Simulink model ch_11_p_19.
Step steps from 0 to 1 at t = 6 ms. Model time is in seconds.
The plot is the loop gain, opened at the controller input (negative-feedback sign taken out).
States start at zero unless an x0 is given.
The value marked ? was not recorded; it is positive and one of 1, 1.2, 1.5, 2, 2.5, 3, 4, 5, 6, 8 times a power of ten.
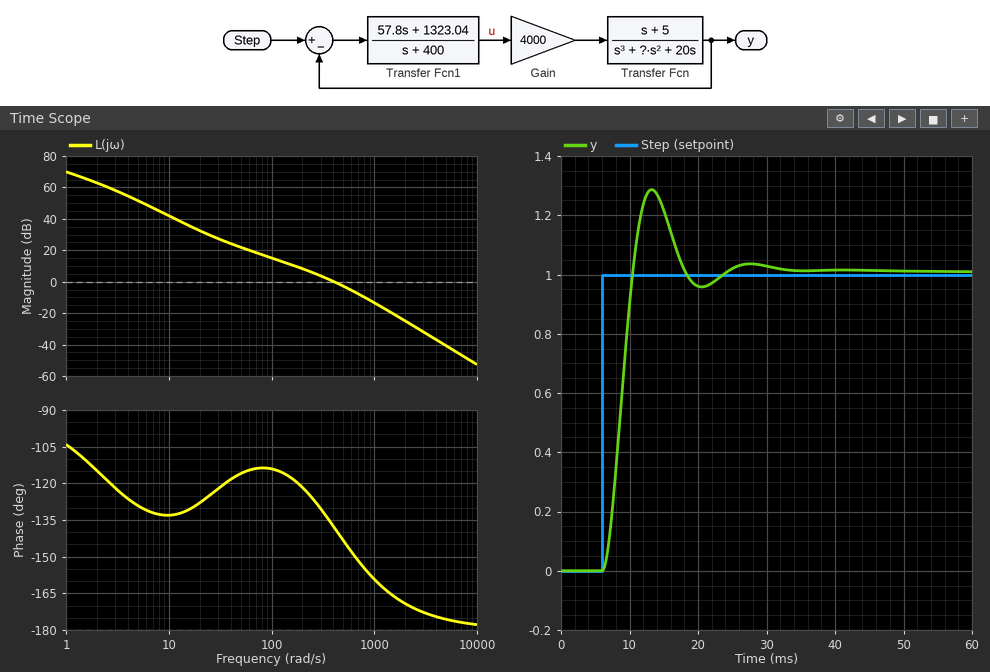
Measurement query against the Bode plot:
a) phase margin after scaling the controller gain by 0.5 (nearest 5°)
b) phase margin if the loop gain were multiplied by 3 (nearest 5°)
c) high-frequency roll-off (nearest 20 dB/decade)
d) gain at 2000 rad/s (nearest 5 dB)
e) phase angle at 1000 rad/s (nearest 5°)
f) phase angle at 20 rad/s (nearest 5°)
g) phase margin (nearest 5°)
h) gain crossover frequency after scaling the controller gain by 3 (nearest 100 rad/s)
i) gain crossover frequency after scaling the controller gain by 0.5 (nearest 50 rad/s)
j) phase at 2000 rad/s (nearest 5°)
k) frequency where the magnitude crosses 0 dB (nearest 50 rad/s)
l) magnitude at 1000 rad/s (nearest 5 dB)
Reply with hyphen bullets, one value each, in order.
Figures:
- 55°
- 25°
- -40 dB/decade
- -25 dB
- -160°
- -130°
- 40°
- 800 rad/s
- 250 rad/s
- -170°
- 400 rad/s
- -15 dB
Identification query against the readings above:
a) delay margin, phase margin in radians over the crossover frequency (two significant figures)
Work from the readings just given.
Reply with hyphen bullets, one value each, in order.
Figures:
- 0.0017 s
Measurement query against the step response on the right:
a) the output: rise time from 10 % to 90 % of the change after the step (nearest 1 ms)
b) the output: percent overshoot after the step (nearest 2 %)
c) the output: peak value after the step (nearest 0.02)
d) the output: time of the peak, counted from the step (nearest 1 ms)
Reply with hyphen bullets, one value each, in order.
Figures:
- 3 ms
- 28 %
- 1.28
- 7 ms
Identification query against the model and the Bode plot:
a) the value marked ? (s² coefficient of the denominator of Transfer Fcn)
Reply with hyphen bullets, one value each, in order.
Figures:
- 10
